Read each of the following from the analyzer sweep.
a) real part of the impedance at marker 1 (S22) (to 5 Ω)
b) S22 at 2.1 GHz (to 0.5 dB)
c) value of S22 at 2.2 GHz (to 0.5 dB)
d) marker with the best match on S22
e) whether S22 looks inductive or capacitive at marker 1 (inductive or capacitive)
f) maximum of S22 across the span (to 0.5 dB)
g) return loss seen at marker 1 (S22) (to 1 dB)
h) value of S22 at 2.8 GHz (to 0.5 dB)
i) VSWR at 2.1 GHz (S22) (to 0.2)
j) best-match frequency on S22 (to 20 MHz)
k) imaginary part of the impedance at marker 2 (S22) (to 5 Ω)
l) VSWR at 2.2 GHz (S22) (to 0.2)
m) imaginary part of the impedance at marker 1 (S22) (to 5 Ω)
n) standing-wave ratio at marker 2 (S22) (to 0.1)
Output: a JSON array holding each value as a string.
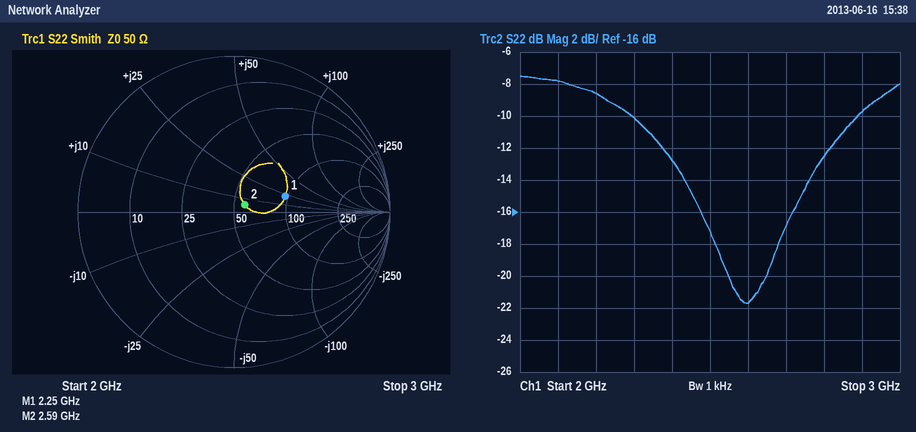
["95 Ω", "-8.0 dB", "-8.5 dB", "marker 2", "inductive", "-7.5 dB", "9 dB", "-12.5 dB", "2.4", "2.60 GHz", "+5 Ω", "2.2", "+20 Ω", "1.2"]
